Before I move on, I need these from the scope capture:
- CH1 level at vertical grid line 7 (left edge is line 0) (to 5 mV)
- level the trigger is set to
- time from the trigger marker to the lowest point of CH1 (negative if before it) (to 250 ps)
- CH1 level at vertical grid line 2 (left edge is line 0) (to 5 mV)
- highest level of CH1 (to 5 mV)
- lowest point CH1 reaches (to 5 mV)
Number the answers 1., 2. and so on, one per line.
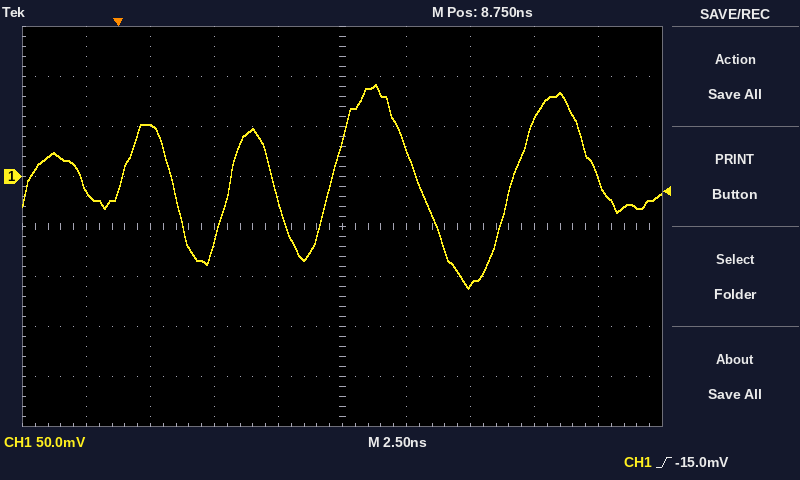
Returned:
1. -110 mV
2. -15.0 mV
3. +13.75 ns
4. 50 mV
5. 90 mV
6. -110 mV
